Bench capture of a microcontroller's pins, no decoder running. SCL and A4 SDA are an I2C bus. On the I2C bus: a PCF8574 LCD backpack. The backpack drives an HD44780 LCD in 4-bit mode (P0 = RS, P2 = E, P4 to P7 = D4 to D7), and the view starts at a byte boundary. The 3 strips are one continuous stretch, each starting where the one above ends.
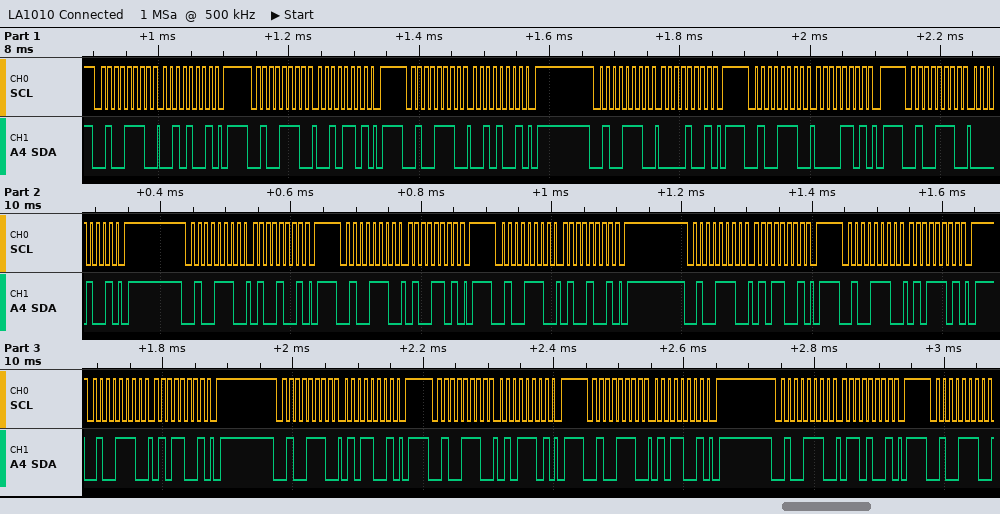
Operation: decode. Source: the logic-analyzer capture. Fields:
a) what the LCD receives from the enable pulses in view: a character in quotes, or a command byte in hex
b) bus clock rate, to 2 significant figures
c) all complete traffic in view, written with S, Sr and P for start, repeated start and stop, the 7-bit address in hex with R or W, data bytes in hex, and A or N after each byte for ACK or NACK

' ' 'E'
100 kHz
S 27W A 29 A P S 27W A 2D A P S 27W A 29 A P S 27W A 09 A P S 27W A 0D A P S 27W A 09 A P S 27W A 49 A P S 27W A 4D A P S 27W A 49 A P S 27W A 59 A P S 27W A 5D A P S 27W A 59 A P S 27W A 59 A P S 27W A 5D A P S 27W A 59 A P S 27W A 69 A P S 27W A
